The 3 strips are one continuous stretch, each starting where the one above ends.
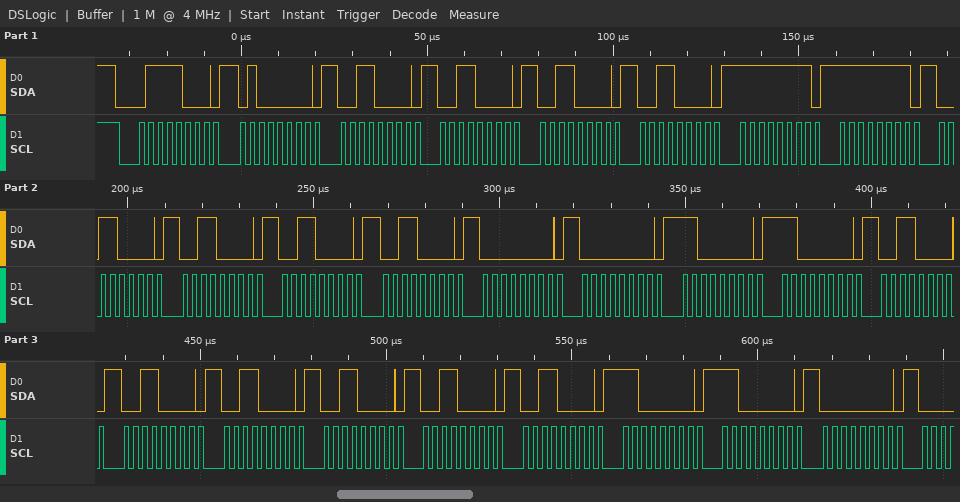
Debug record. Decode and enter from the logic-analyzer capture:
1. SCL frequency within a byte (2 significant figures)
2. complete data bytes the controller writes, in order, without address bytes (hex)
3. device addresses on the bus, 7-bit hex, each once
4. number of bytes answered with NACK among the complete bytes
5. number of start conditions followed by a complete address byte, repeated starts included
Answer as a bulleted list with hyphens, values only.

- 400 kHz
- 40 30 30 30 30 FF FF 30 30 30 30 00 00 C0 C0 30 30 30 30 30 30 C0 C0 00
- 0x3C
- 0
- 1
